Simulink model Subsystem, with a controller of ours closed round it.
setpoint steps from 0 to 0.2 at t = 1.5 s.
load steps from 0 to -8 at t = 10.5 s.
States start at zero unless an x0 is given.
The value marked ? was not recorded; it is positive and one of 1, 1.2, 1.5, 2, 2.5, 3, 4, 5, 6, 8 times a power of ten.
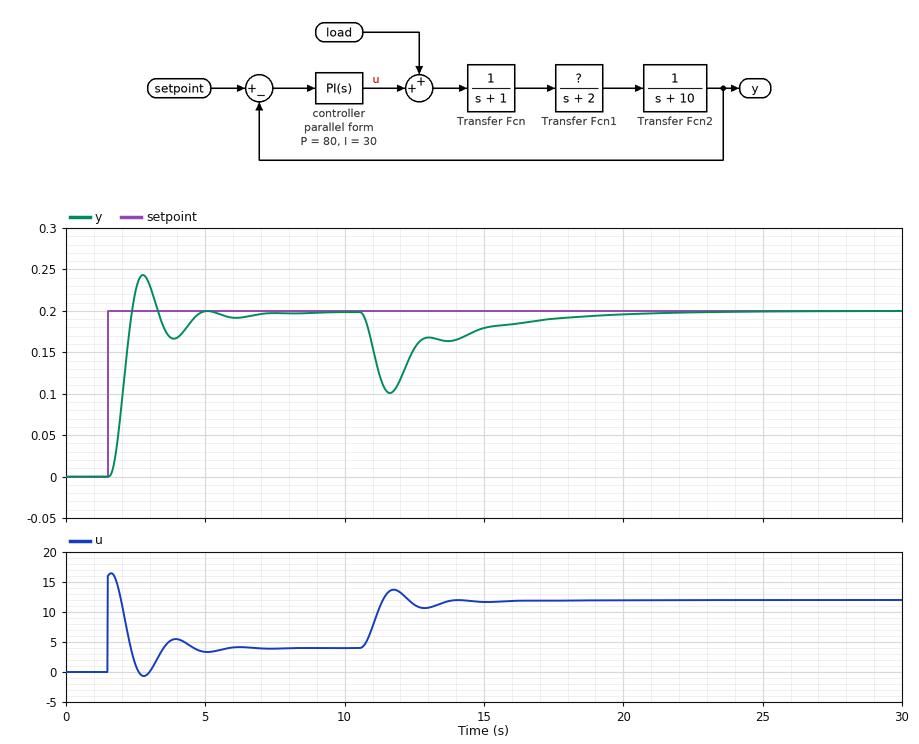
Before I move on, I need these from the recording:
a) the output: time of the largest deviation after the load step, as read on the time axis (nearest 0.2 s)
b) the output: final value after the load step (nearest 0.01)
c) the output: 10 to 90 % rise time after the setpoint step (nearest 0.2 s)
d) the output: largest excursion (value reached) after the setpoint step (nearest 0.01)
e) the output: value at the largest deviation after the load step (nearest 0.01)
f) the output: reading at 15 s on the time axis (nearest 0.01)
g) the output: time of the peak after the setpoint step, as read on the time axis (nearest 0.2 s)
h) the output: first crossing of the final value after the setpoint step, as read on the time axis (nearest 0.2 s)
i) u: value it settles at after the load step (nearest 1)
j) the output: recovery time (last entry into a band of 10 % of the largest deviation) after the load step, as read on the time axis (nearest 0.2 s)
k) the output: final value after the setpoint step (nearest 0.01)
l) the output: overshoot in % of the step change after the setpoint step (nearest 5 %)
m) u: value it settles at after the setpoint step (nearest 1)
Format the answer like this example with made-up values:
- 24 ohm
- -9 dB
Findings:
- 11.6 s
- 0.20
- 0.6 s
- 0.24
- 0.10
- 0.18
- 2.8 s
- 2.4 s
- 12
- 17.4 s
- 0.20
- 20 %
- 4
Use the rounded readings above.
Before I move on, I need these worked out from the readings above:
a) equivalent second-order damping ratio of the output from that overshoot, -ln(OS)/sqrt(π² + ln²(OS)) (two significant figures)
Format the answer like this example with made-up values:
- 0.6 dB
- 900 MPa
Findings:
- 0.46
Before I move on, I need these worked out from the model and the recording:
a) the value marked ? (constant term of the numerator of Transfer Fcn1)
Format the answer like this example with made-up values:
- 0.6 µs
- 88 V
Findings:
- 1
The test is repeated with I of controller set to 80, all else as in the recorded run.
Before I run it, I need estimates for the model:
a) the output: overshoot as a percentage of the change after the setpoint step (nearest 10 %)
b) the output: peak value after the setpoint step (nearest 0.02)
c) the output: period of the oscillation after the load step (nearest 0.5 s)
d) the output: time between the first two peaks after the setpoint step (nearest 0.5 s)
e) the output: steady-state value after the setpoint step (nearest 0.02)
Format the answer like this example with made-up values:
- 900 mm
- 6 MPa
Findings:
- 50 %
- 0.30
- 2.5 s
- 2.5 s
- 0.20
